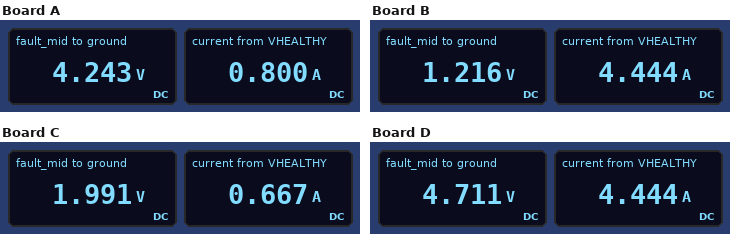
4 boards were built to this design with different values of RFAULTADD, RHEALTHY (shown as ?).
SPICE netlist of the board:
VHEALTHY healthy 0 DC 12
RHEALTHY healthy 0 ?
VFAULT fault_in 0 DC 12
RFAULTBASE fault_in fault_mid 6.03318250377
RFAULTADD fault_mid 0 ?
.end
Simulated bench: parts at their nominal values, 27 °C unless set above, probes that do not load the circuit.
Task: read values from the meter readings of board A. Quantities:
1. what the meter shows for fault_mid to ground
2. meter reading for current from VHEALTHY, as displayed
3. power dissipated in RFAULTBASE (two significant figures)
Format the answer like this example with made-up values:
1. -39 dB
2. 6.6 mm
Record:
1. 4.243 V
2. 0.800 A
3. 10 W
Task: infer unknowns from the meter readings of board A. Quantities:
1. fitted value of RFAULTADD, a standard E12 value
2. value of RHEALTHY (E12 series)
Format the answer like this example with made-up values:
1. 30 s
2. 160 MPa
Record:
1. 3.3 Ω
2. 15 Ω
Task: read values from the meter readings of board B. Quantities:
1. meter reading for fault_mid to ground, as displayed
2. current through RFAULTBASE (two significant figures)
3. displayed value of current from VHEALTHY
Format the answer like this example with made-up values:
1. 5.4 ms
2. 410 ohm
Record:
1. 1.216 V
2. 1.8 A
3. 4.444 A
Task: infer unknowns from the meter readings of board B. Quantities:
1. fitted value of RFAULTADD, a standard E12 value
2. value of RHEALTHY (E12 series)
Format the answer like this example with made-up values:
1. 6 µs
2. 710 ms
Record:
1. 0.68 Ω
2. 2.7 Ω
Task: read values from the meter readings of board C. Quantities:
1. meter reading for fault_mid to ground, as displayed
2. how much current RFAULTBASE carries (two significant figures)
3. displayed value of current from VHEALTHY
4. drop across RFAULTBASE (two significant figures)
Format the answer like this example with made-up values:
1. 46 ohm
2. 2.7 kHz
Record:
1. 1.991 V
2. 1.7 A
3. 0.667 A
4. 10 V
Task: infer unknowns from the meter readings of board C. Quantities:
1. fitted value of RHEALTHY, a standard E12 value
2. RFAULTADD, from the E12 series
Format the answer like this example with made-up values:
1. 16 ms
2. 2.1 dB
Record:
1. 18 Ω
2. 1.2 Ω
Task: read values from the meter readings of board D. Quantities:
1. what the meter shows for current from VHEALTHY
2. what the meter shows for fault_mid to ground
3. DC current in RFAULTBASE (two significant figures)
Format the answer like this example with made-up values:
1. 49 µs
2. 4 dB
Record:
1. 4.444 A
2. 4.711 V
3. 1.2 A
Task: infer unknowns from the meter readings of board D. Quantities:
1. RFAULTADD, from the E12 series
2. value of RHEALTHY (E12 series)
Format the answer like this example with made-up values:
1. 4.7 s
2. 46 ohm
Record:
1. 3.9 Ω
2. 2.7 Ω
